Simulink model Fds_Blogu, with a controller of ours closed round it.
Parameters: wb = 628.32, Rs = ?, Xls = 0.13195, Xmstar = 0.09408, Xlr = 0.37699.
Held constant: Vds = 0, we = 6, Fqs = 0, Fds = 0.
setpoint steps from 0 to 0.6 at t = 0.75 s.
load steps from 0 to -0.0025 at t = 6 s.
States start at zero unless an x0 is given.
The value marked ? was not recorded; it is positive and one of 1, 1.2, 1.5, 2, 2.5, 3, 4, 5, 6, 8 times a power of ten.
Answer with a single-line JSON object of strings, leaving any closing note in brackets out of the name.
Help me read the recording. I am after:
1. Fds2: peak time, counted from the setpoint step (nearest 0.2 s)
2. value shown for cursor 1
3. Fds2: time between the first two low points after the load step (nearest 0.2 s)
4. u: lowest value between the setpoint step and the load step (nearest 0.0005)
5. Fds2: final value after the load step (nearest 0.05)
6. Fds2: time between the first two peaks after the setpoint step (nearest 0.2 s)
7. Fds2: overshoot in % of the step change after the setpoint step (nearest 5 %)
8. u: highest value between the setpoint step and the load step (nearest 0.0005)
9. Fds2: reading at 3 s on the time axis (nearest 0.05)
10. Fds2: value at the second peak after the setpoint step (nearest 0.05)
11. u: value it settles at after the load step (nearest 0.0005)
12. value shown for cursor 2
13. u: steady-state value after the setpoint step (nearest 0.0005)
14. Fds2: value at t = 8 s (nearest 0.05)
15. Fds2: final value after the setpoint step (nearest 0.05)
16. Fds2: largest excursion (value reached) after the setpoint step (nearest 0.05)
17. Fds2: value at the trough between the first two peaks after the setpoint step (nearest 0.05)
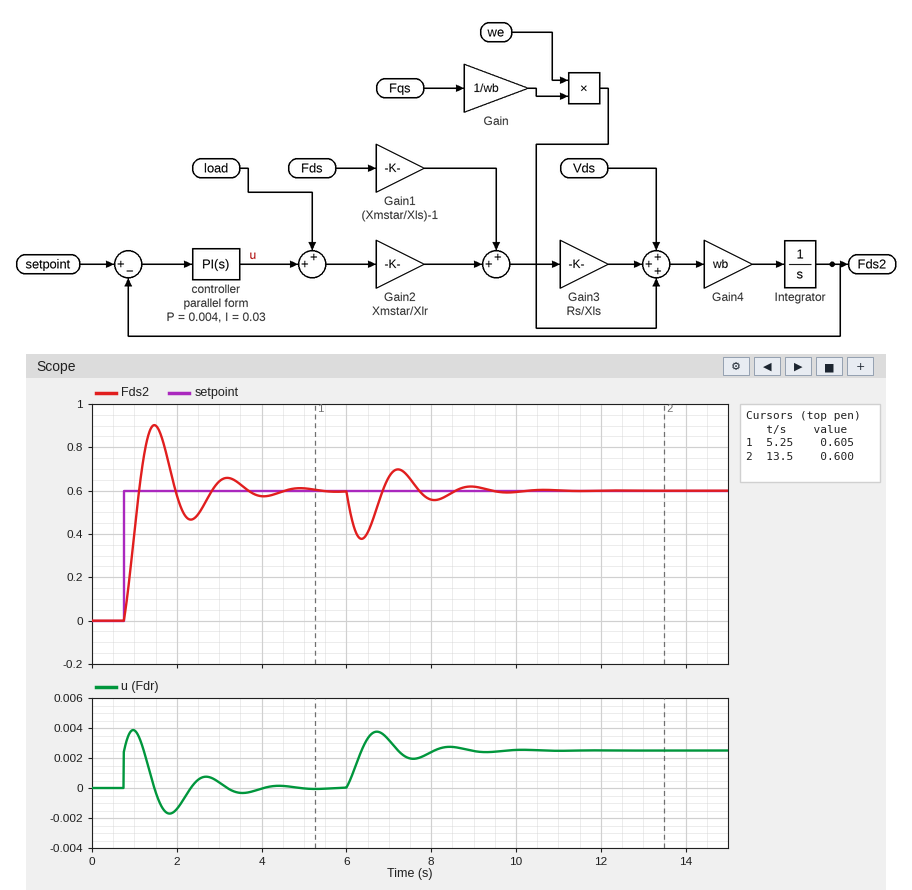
{"Fds2: peak time, counted from the setpoint step": "0.8 s", "value shown for cursor 1": "0.605", "Fds2: time between the first two low points after the load step": "1.8 s", "u: lowest value between the setpoint step and the load step": "-0.0015", "Fds2: final value after the load step": "0.60", "Fds2: time between the first two peaks after the setpoint step": "1.8 s", "Fds2: overshoot in % of the step change after the setpoint step": "50 %", "u: highest value between the setpoint step and the load step": "0.0040", "Fds2: reading at 3 s on the time axis": "0.65", "Fds2: value at the second peak after the setpoint step": "0.65", "u: value it settles at after the load step": "0.0025", "value shown for cursor 2": "0.600", "u: steady-state value after the setpoint step": "0.0000", "Fds2: value at t = 8 s": "0.55", "Fds2: final value after the setpoint step": "0.60", "Fds2: largest excursion (value reached) after the setpoint step": "0.90", "Fds2: value at the trough between the first two peaks after the setpoint step": "0.45"}
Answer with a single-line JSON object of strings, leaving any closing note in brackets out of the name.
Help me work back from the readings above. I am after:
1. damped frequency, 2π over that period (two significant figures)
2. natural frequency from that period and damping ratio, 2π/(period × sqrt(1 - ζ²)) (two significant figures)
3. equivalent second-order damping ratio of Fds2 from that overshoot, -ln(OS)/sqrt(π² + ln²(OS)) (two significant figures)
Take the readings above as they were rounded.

{"damped frequency, 2π over that period": "3.5 rad/s", "natural frequency from that period and damping ratio, 2π/(period × sqrt(1 - ζ²))": "3.6 rad/s", "equivalent second-order damping ratio of Fds2 from that overshoot, -ln(OS)/sqrt(π² + ln²(OS))": "0.22"}
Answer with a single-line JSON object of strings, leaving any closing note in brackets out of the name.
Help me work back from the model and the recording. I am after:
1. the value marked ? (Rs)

{"the value marked ?": "0.4"}
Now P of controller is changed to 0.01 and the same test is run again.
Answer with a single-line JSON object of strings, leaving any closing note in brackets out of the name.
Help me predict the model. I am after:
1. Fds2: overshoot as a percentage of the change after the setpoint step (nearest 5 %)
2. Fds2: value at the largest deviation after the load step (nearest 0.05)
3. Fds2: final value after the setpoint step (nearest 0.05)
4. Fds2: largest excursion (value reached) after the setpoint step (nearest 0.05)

{"Fds2: overshoot as a percentage of the change after the setpoint step": "25 %", "Fds2: value at the largest deviation after the load step": "0.45", "Fds2: final value after the setpoint step": "0.60", "Fds2: largest excursion (value reached) after the setpoint step": "0.75"}
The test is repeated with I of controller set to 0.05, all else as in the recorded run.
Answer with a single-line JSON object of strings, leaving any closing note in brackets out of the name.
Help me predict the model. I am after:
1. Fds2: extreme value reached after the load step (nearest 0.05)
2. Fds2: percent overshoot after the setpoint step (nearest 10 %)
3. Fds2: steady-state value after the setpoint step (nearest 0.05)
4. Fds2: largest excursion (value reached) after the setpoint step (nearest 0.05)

{"Fds2: extreme value reached after the load step": "0.40", "Fds2: percent overshoot after the setpoint step": "60 %", "Fds2: steady-state value after the setpoint step": "0.60", "Fds2: largest excursion (value reached) after the setpoint step": "0.95"}
